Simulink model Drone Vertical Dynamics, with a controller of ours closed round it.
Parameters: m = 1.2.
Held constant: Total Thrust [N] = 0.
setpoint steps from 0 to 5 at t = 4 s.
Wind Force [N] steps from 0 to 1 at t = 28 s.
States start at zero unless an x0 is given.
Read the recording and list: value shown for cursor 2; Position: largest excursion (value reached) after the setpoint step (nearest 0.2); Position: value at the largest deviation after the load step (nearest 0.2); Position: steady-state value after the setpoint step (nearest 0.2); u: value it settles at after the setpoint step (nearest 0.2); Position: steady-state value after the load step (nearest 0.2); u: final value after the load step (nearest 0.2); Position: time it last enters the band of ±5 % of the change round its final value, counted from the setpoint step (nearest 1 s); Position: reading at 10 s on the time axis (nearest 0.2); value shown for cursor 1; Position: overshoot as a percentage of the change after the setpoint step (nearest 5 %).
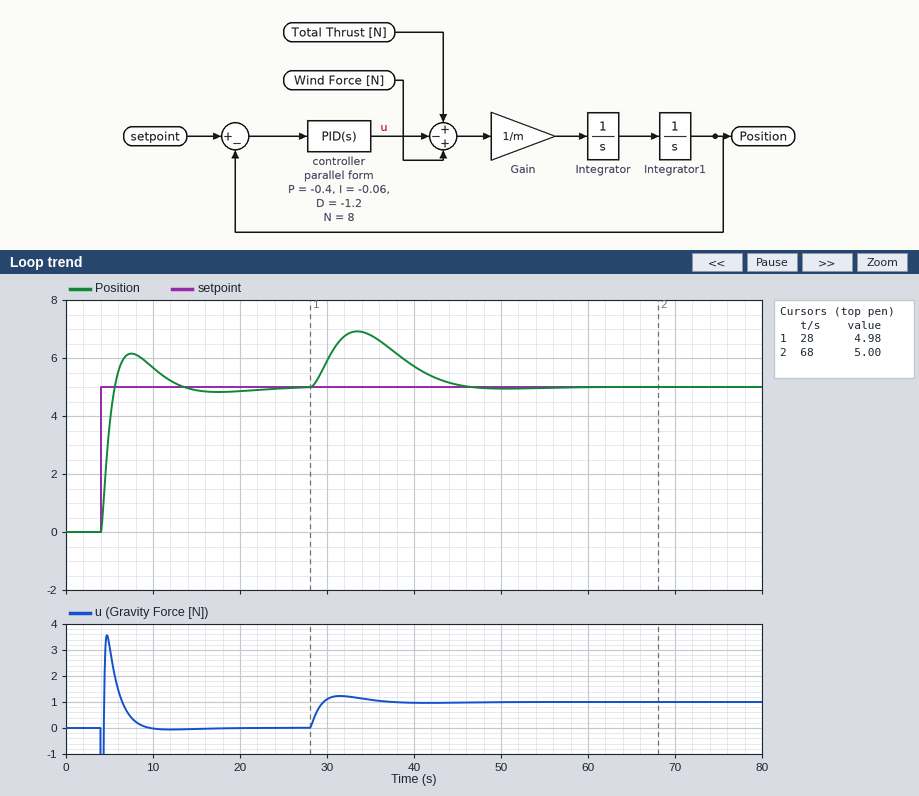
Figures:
5.00
6.2
7.0
5.0
0.0
5.0
1.0
8 s
5.6
4.98
25 %
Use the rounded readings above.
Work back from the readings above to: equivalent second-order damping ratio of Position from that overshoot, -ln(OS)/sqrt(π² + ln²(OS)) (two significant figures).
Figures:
0.40
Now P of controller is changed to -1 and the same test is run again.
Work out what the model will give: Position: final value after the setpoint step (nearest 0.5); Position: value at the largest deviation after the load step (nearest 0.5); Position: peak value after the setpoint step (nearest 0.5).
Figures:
5.0
6.0
6.5
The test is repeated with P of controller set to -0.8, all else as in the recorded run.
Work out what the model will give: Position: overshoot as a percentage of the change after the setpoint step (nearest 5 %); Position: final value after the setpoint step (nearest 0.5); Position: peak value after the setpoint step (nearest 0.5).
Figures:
30 %
5.0
6.5
